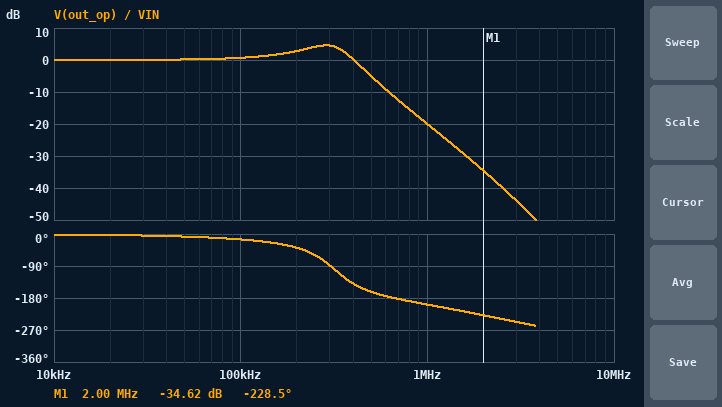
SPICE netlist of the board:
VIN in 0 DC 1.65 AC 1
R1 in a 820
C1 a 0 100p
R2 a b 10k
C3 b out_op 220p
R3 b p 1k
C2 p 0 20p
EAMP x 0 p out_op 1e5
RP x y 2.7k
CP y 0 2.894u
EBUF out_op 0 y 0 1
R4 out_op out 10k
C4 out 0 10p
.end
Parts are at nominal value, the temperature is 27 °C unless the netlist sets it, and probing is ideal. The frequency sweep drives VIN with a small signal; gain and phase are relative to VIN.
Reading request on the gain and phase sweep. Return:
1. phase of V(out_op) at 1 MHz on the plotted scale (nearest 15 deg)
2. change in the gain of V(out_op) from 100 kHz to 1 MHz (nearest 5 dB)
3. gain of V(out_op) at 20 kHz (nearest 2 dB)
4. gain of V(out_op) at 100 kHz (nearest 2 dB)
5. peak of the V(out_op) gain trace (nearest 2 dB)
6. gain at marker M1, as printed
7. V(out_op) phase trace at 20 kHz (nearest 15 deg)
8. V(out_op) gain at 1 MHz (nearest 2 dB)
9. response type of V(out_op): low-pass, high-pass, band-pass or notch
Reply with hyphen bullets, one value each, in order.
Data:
- -195 deg
- -20 dB
- 0 dB
- 0 dB
- 4 dB
- -34.62 dB
- 0 deg
- -20 dB
- low-pass
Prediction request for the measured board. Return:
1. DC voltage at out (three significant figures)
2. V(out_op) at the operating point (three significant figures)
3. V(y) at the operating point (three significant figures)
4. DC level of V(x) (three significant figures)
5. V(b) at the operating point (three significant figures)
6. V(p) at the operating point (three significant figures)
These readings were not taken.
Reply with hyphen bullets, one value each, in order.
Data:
- 1.65 V
- 1.65 V
- 1.65 V
- 1.65 V
- 1.65 V
- 1.65 V
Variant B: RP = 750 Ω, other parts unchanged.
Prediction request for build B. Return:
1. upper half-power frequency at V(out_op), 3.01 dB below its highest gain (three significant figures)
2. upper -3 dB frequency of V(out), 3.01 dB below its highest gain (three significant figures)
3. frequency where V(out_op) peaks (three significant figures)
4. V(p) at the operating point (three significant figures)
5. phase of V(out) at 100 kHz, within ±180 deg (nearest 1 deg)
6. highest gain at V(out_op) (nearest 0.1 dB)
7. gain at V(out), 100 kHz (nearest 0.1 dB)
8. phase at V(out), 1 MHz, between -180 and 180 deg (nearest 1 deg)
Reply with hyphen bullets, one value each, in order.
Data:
- 588 kHz
- 578 kHz
- 408 kHz
- 1.65 V
- -16 deg
- 2.6 dB
- 0.2 dB
- 147 deg
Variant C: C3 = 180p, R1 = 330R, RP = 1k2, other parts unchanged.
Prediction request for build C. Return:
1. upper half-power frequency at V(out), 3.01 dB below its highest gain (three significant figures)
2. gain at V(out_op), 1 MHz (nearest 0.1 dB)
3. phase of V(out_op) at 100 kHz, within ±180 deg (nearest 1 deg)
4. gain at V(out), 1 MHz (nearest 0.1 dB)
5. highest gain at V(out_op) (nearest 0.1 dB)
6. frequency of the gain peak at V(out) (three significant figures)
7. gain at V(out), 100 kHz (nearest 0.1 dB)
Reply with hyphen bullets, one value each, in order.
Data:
- 570 kHz
- -11.3 dB
- -11 deg
- -12.7 dB
- 3.0 dB
- 402 kHz
- 0.2 dB
